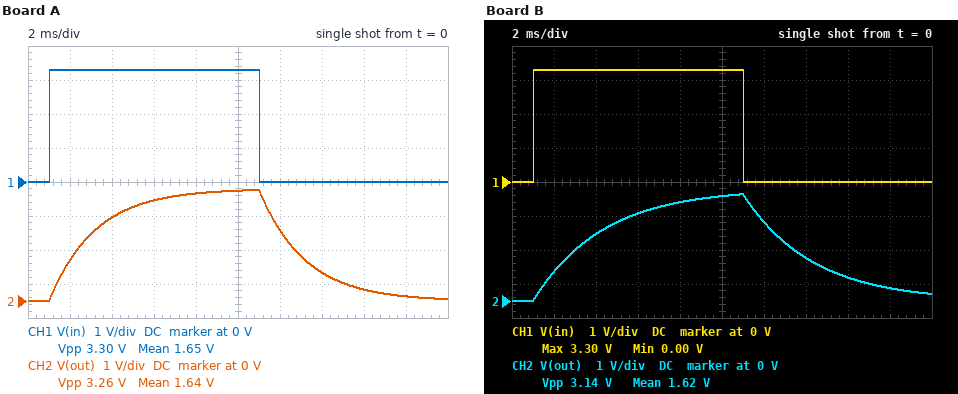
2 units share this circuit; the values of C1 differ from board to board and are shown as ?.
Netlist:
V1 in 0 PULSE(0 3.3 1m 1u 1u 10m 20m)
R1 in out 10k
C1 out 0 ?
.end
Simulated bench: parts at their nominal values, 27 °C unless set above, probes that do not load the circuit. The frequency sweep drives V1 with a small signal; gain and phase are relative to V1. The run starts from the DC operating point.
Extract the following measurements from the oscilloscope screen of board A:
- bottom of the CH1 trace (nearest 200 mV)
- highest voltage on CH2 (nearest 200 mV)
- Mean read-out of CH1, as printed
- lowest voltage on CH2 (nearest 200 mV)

0 V
3.2 V
1.65 V
0 V
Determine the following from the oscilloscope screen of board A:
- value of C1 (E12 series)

220 nF
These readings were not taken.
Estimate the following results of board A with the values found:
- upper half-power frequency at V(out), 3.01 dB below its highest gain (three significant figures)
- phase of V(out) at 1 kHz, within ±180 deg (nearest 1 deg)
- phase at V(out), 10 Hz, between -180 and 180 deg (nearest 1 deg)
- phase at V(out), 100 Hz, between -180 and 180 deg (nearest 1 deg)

72.3 Hz
-86 deg
-8 deg
-54 deg
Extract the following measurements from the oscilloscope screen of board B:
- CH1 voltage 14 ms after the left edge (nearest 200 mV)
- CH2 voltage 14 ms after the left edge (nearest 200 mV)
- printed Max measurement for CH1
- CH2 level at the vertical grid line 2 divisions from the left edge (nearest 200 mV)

0 V
1.2 V
3.30 V
2.0 V
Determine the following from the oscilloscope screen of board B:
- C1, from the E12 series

330 nF
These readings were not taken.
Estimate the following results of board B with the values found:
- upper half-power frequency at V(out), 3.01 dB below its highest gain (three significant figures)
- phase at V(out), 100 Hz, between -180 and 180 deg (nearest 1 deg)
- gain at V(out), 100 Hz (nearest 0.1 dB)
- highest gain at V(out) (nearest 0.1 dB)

48.2 Hz
-64 deg
-7.2 dB
0 dB
